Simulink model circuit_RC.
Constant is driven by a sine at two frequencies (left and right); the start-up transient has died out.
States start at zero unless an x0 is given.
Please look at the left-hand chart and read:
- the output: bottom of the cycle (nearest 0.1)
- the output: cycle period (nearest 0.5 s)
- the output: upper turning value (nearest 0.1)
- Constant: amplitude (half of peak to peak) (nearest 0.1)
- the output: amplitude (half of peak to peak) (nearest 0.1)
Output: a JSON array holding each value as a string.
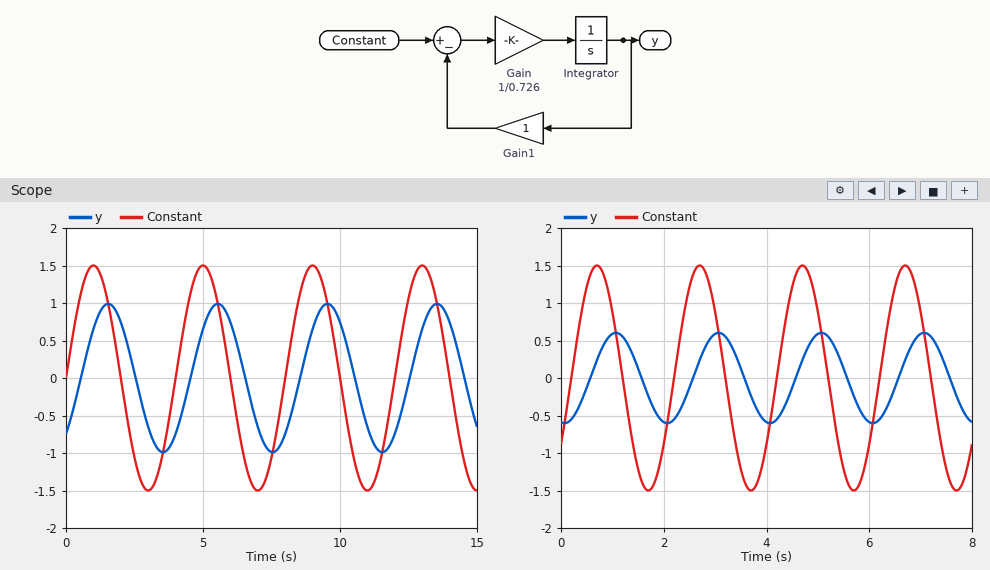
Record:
["-1.0", "4.0 s", "1.0", "1.5", "1.0"]
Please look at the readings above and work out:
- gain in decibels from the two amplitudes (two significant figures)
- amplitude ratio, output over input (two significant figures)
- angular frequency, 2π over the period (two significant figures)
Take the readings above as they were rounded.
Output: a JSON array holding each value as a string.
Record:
["-3.5 dB", "0.67", "1.6 rad/s"]
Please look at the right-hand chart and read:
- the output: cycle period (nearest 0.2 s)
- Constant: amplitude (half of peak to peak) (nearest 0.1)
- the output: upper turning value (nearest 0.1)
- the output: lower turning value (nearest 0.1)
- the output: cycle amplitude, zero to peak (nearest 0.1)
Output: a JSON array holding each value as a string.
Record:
["2.0 s", "1.5", "0.6", "-0.6", "0.6"]
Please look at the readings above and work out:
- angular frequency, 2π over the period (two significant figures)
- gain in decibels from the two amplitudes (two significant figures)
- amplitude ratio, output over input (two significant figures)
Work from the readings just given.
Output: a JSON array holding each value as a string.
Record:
["3.1 rad/s", "-8.0 dB", "0.40"]
